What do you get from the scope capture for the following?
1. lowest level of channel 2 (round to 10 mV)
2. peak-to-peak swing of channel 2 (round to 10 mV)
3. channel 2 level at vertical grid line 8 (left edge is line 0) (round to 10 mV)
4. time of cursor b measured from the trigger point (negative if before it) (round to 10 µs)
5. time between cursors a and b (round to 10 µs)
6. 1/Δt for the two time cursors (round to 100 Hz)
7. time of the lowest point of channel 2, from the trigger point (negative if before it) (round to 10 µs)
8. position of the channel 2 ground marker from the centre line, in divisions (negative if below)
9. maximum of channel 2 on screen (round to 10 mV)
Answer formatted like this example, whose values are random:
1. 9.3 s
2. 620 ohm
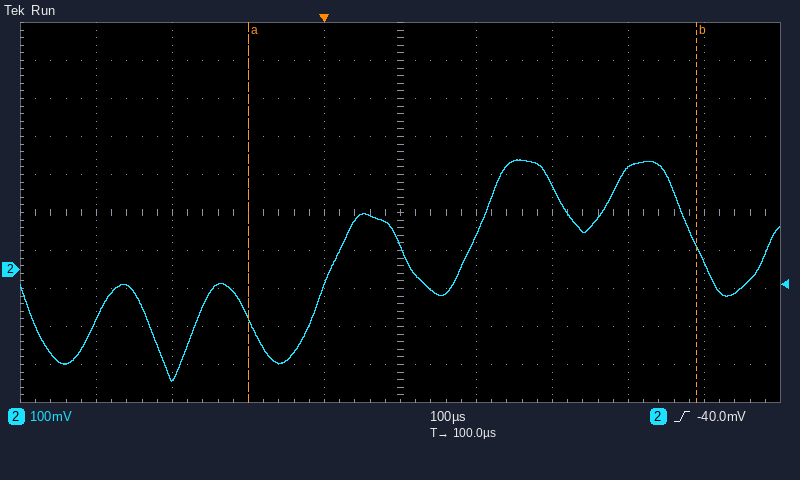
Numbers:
1. -290 mV
2. 580 mV
3. 270 mV
4. +490 µs
5. 590 µs
6. 1.7 kHz
7. -200 µs
8. -1.5 div
9. 290 mV
